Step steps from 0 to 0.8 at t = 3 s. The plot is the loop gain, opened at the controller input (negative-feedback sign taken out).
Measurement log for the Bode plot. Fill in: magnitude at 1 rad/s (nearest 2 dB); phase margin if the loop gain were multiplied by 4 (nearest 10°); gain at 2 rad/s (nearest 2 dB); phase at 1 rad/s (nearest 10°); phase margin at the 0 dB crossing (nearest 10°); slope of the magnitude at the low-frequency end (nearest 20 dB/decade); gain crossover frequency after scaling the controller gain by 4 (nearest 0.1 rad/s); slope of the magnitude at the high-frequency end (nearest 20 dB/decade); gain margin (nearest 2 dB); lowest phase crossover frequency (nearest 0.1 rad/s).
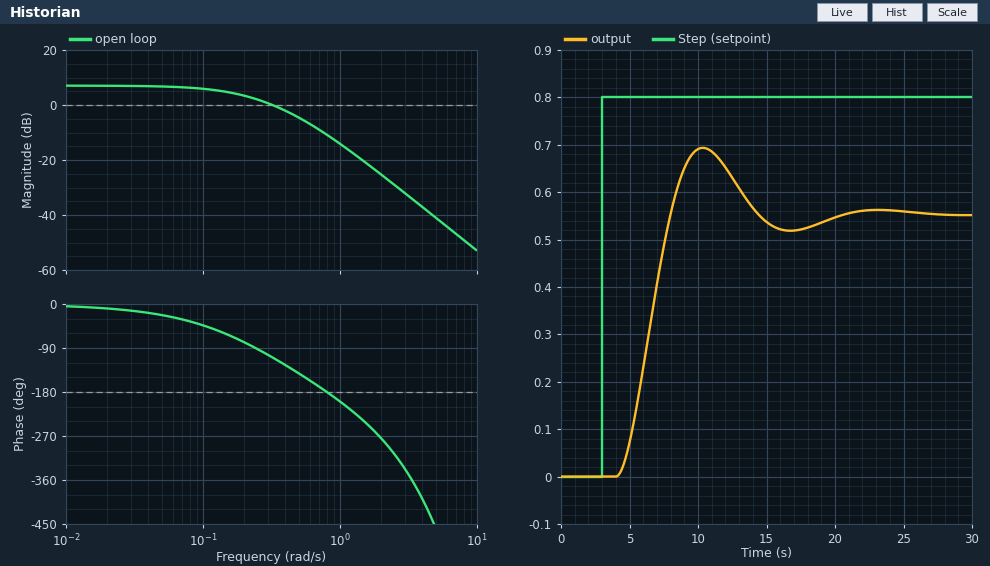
-14 dB
-10°
-26 dB
-200°
70°
0 dB/decade
0.9 rad/s
-40 dB/decade
10 dB
0.8 rad/s
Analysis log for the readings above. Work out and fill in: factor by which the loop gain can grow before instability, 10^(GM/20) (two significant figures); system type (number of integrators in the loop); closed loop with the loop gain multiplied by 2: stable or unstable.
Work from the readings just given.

3.2
0
stable
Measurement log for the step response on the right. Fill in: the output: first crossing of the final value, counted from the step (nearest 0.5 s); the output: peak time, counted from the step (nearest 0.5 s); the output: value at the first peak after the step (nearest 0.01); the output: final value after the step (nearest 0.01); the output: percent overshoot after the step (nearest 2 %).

5.0 s
7.5 s
0.69
0.55
26 %
